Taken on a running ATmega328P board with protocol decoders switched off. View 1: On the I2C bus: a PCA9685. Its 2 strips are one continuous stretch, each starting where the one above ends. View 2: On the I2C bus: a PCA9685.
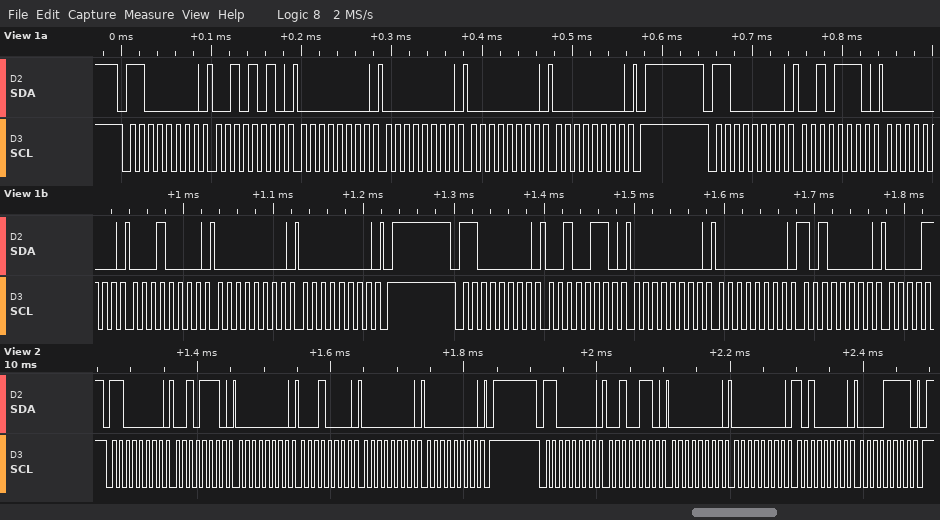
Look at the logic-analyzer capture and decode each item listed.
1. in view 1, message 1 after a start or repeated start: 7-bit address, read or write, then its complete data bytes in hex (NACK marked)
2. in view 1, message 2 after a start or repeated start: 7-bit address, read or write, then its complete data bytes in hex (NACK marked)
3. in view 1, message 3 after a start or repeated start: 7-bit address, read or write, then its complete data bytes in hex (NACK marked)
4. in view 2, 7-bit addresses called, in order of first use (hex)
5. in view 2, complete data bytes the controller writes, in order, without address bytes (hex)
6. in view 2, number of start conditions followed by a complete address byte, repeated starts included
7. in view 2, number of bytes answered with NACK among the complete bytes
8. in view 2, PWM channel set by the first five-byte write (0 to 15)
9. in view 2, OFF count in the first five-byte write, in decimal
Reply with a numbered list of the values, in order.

1. 0x60 write: 2A 00 00 00 00
2. 0x60 write: 2E 00 10 00 00
3. 0x60 write: 26 00 00 A0
4. 0x60
5. 2E 00 10 00 00 26 00 00 A0 0F
6. 2
7. 0
8. 10
9. 0
